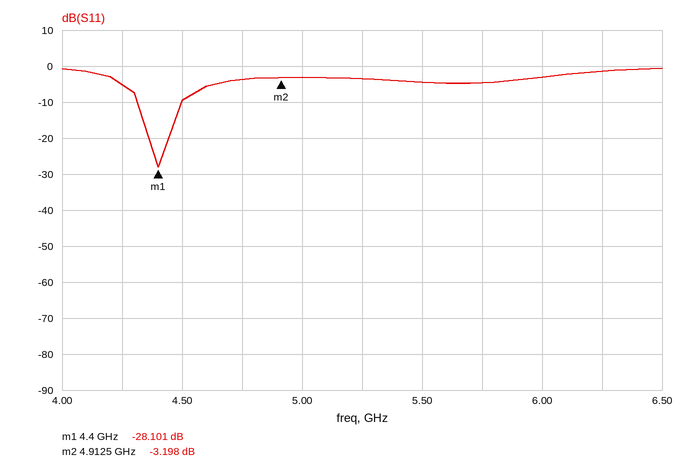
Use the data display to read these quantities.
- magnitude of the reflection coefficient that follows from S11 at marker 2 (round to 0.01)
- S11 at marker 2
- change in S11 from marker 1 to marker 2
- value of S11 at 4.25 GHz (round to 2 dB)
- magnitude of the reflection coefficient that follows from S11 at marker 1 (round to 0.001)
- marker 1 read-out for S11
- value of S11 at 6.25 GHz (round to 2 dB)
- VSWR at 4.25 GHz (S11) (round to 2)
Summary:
0.69
-3.198 dB
24.903 dB
-6 dB
0.039
-28.101 dB
-2 dB
4
